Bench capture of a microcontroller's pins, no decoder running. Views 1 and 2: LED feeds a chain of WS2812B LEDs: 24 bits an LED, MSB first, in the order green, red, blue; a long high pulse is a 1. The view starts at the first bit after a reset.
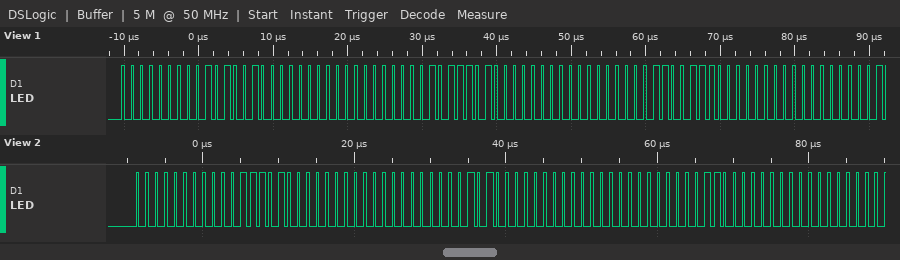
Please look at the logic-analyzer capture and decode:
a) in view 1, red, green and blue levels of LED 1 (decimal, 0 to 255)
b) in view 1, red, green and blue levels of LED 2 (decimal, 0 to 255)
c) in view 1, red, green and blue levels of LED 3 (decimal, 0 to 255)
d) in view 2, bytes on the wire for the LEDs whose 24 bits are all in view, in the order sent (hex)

82, 0, 0
93, 0, 0
103, 0, 0
00 1D 00 00 14 00 00 0C 00
